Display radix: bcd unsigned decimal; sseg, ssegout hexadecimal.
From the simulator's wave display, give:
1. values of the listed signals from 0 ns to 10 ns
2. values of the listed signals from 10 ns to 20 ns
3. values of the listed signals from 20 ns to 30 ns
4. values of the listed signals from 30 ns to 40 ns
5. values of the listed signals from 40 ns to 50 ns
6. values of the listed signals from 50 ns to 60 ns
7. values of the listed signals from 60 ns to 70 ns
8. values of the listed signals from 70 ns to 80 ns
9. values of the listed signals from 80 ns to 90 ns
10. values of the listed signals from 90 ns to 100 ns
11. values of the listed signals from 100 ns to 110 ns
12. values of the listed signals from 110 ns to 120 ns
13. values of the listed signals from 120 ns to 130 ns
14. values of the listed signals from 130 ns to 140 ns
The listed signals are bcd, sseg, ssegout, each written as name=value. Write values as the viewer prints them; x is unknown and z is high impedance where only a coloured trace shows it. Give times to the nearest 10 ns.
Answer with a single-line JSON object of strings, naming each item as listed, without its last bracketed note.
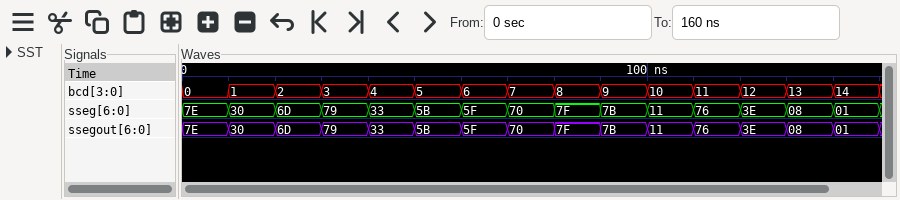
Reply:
{"values of the listed signals from 0 ns to 10 ns": "bcd=0, sseg=7E, ssegout=7E", "values of the listed signals from 10 ns to 20 ns": "bcd=1, sseg=30, ssegout=30", "values of the listed signals from 20 ns to 30 ns": "bcd=2, sseg=6D, ssegout=6D", "values of the listed signals from 30 ns to 40 ns": "bcd=3, sseg=79, ssegout=79", "values of the listed signals from 40 ns to 50 ns": "bcd=4, sseg=33, ssegout=33", "values of the listed signals from 50 ns to 60 ns": "bcd=5, sseg=5B, ssegout=5B", "values of the listed signals from 60 ns to 70 ns": "bcd=6, sseg=5F, ssegout=5F", "values of the listed signals from 70 ns to 80 ns": "bcd=7, sseg=70, ssegout=70", "values of the listed signals from 80 ns to 90 ns": "bcd=8, sseg=7F, ssegout=7F", "values of the listed signals from 90 ns to 100 ns": "bcd=9, sseg=7B, ssegout=7B", "values of the listed signals from 100 ns to 110 ns": "bcd=10, sseg=11, ssegout=11", "values of the listed signals from 110 ns to 120 ns": "bcd=11, sseg=76, ssegout=76", "values of the listed signals from 120 ns to 130 ns": "bcd=12, sseg=3E, ssegout=3E", "values of the listed signals from 130 ns to 140 ns": "bcd=13, sseg=08, ssegout=08"}
